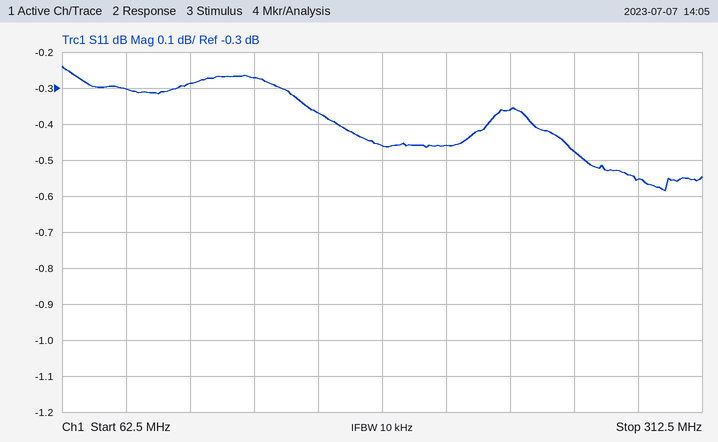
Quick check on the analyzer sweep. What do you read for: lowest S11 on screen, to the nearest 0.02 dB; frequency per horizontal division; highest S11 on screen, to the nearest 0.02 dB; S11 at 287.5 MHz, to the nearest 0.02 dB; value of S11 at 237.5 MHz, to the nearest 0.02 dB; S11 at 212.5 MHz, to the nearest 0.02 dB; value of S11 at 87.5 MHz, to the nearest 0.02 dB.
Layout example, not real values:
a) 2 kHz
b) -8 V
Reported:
a) -0.58 dB
b) 25 MHz
c) -0.24 dB
d) -0.56 dB
e) -0.36 dB
f) -0.46 dB
g) -0.30 dB
